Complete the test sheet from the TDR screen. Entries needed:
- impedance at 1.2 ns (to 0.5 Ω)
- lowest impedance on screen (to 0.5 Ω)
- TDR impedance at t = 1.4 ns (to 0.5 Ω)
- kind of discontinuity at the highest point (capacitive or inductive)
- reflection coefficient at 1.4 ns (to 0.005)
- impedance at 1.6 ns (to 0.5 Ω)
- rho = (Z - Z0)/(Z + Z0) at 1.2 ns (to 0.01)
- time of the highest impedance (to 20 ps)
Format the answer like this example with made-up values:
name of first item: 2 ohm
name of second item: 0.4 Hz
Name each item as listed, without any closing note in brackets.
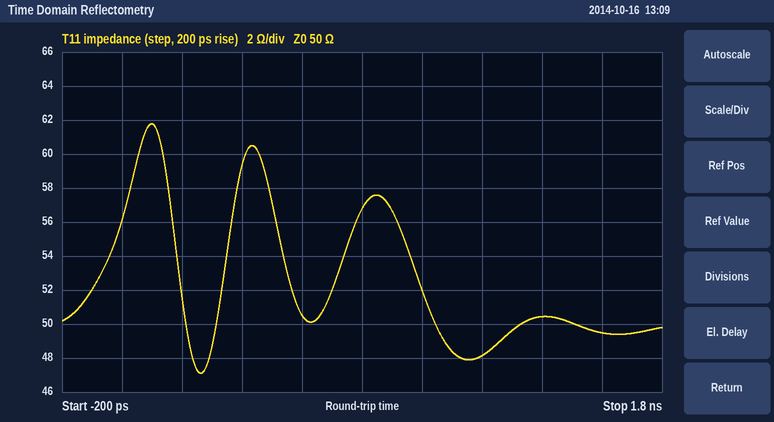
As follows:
impedance at 1.2 ns: 48.0 Ω
lowest impedance on screen: 47.0 Ω
TDR impedance at t = 1.4 ns: 50.5 Ω
kind of discontinuity at the highest point: inductive
reflection coefficient at 1.4 ns: +0.005
impedance at 1.6 ns: 49.5 Ω
rho = (Z - Z0)/(Z + Z0) at 1.2 ns: -0.02
time of the highest impedance: 100 ps
